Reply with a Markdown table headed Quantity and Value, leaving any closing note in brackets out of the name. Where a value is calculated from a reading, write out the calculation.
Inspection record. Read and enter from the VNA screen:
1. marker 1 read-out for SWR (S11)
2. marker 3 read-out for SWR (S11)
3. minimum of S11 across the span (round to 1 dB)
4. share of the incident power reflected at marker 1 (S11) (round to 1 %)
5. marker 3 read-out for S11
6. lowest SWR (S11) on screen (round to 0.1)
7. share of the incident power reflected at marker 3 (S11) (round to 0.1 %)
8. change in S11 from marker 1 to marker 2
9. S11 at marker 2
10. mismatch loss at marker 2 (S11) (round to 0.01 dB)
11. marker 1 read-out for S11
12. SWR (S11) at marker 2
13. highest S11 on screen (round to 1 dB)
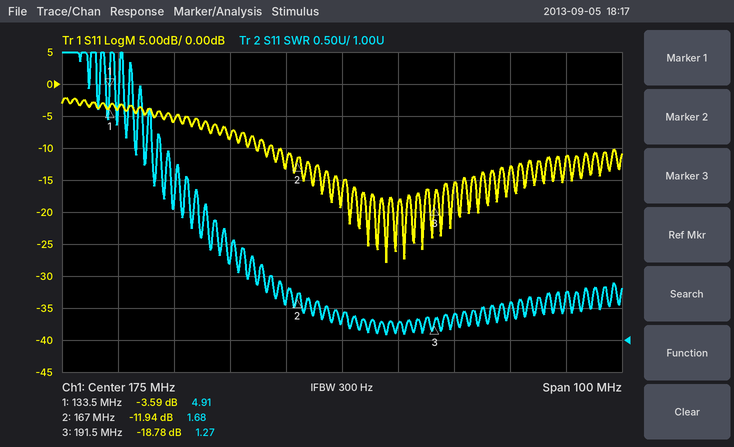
| Quantity | Value |
|---|---|
| marker 1 read-out for SWR | 4.91 |
| marker 3 read-out for SWR | 1.27 |
| minimum of S11 across the span | -28 dB |
| share of the incident power reflected at marker 1 (S11) | 10^(-3.59/10) ≈ 44 % |
| marker 3 read-out for S11 | -18.78 dB |
| lowest SWR (S11) on screen | 1.1 |
| share of the incident power reflected at marker 3 (S11) | 10^(-18.78/10) ≈ 1.3 % |
| change in S11 from marker 1 to marker 2 | -11.94 − (-3.59) = -8.35 dB |
| S11 at marker 2 | -11.94 dB |
| mismatch loss at marker 2 (S11) | −10 log10(1 − 10^(-11.94/10)) ≈ 0.29 dB |
| marker 1 read-out for S11 | -3.59 dB |
| SWR (S11) at marker 2 | 1.68 |
| highest S11 on screen | -2 dB |
